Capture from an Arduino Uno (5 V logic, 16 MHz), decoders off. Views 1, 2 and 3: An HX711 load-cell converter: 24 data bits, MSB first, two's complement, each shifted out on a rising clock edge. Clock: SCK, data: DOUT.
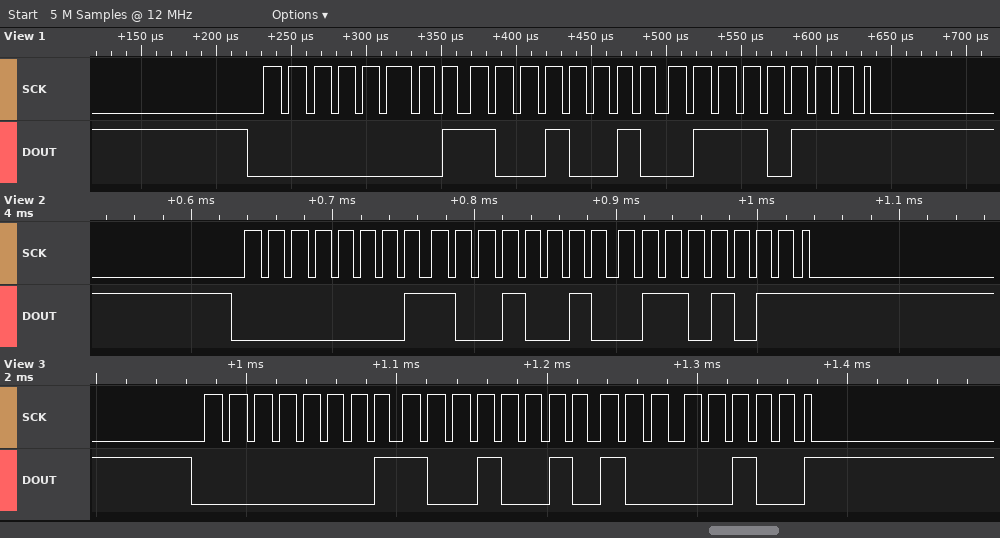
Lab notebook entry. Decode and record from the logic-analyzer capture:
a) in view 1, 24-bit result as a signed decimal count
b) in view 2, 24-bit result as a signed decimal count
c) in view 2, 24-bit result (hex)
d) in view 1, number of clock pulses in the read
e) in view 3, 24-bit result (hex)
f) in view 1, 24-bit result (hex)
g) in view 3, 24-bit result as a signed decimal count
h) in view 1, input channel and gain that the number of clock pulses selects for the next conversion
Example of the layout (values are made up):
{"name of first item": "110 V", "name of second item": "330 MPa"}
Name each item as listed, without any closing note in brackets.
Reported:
{"in view 1, 24-bit result as a signed decimal count": "103031", "in view 2, 24-bit result as a signed decimal count": "103019", "in view 2, 24-bit result": "0x01926B", "in view 1, number of clock pulses in the read": "25", "in view 3, 24-bit result": "0x019284", "in view 1, 24-bit result": "0x019277", "in view 3, 24-bit result as a signed decimal count": "103044", "in view 1, input channel and gain that the number of clock pulses selects for the next conversion": "channel A, gain 128"}
